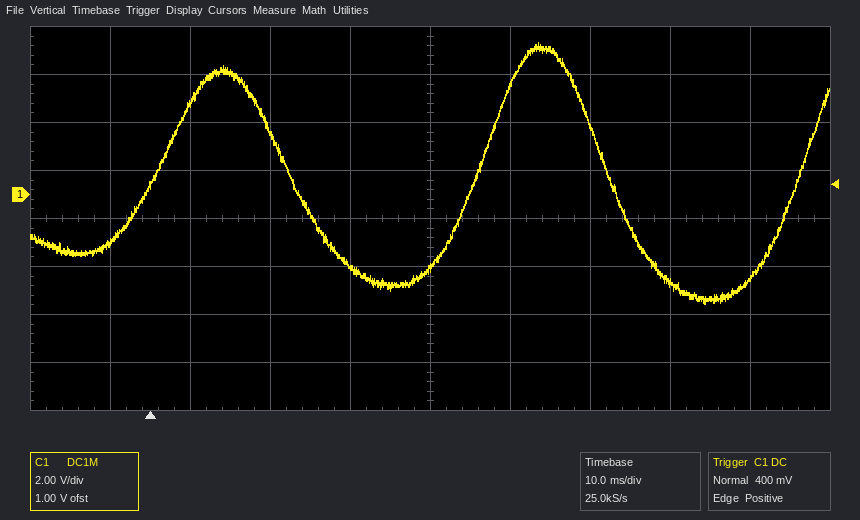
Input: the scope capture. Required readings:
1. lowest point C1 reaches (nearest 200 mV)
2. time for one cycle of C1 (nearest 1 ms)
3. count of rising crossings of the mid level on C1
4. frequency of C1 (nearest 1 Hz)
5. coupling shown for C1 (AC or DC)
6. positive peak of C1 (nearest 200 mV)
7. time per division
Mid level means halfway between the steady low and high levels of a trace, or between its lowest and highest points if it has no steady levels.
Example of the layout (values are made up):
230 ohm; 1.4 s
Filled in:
-4.6 V; 40 ms; 3; 25 Hz; DC; 6.4 V; 10 ms
